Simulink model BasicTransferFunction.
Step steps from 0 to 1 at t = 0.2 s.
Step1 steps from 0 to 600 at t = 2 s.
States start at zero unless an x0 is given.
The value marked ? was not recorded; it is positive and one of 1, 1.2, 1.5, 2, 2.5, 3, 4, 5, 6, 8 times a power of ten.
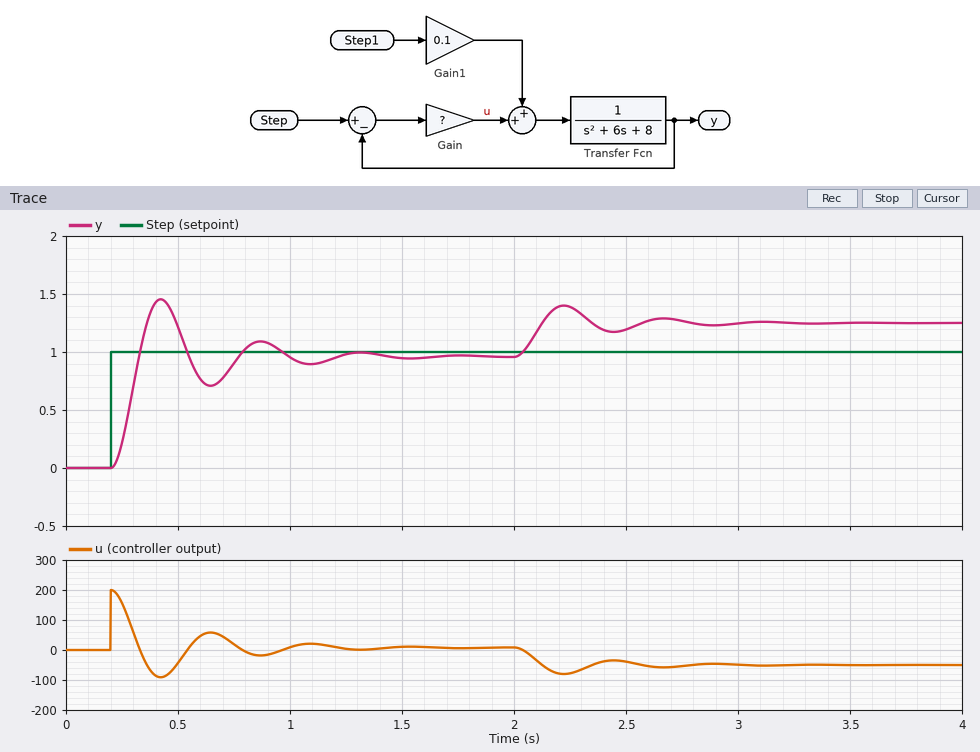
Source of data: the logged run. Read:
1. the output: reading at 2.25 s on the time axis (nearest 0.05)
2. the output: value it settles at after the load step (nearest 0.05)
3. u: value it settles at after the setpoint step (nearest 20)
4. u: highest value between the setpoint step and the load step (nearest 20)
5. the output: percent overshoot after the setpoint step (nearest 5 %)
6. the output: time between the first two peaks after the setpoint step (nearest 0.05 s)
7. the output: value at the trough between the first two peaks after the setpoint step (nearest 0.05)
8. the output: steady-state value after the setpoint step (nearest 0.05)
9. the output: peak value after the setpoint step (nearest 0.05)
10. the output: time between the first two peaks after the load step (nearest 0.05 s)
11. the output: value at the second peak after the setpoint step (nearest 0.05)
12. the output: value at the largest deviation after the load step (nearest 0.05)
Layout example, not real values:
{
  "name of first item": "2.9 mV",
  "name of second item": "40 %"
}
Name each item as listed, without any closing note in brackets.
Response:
{
  "the output: reading at 2.25 s on the time axis": "1.40",
  "the output: value it settles at after the load step": "1.25",
  "u: value it settles at after the setpoint step": "0",
  "u: highest value between the setpoint step and the load step": "200",
  "the output: percent overshoot after the setpoint step": "50 %",
  "the output: time between the first two peaks after the setpoint step": "0.45 s",
  "the output: value at the trough between the first two peaks after the setpoint step": "0.70",
  "the output: steady-state value after the setpoint step": "0.95",
  "the output: peak value after the setpoint step": "1.45",
  "the output: time between the first two peaks after the load step": "0.45 s",
  "the output: value at the second peak after the setpoint step": "1.10",
  "the output: value at the largest deviation after the load step": "1.40"
}
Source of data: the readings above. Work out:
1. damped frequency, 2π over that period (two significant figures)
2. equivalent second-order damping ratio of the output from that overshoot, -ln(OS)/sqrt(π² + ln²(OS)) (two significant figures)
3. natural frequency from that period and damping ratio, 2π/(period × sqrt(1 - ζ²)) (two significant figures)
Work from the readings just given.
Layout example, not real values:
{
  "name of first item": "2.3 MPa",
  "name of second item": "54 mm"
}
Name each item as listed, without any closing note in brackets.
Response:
{
  "damped frequency, 2π over that period": "14 rad/s",
  "equivalent second-order damping ratio of the output from that overshoot, -ln(OS)/sqrt(π² + ln²(OS))": "0.22",
  "natural frequency from that period and damping ratio, 2π/(period × sqrt(1 - ζ²))": "14 rad/s"
}
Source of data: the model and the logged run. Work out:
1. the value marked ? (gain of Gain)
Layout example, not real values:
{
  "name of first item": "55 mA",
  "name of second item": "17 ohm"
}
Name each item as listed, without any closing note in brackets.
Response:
{
  "the value marked ?": "200"
}
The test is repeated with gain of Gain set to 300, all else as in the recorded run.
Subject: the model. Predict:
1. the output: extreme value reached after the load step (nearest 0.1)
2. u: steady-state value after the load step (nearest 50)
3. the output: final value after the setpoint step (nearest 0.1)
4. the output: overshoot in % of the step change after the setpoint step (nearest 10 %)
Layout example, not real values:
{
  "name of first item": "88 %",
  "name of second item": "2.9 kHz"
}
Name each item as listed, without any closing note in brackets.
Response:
{
  "the output: extreme value reached after the load step": "1.3",
  "u: steady-state value after the load step": "-50",
  "the output: final value after the setpoint step": "1.0",
  "the output: overshoot in % of the step change after the setpoint step": "60 %"
}
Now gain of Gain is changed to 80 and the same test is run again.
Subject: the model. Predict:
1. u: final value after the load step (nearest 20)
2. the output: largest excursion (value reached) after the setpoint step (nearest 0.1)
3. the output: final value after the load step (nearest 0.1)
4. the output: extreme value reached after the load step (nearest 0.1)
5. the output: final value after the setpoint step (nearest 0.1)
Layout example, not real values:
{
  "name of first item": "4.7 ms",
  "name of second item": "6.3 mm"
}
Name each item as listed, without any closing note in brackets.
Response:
{
  "u: final value after the load step": "-40",
  "the output: largest excursion (value reached) after the setpoint step": "1.2",
  "the output: final value after the load step": "1.6",
  "the output: extreme value reached after the load step": "1.8",
  "the output: final value after the setpoint step": "0.9"
}
